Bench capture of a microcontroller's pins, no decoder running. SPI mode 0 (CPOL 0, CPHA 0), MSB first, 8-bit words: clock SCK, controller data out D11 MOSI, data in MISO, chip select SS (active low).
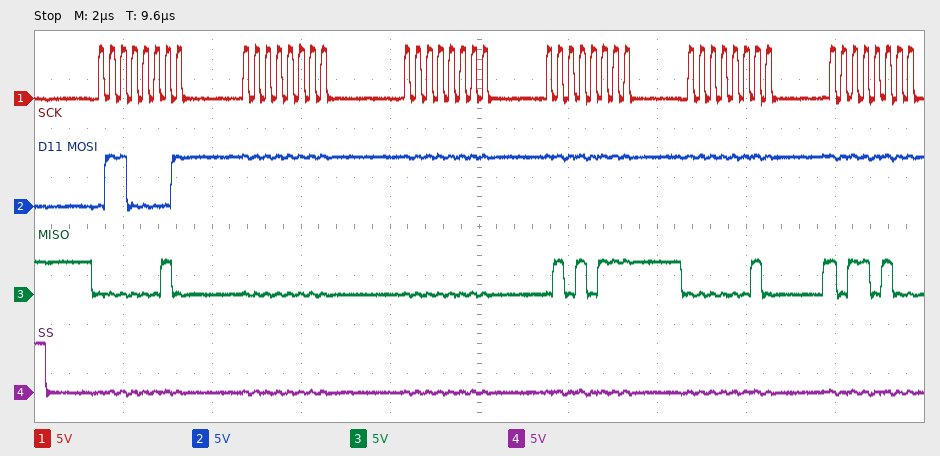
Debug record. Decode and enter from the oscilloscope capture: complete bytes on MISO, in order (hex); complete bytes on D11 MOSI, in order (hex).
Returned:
0x02 0x00 0x00 0x57 0x02 0xB4
0x61 0xFF 0xFF 0xFF 0xFF 0xFF
